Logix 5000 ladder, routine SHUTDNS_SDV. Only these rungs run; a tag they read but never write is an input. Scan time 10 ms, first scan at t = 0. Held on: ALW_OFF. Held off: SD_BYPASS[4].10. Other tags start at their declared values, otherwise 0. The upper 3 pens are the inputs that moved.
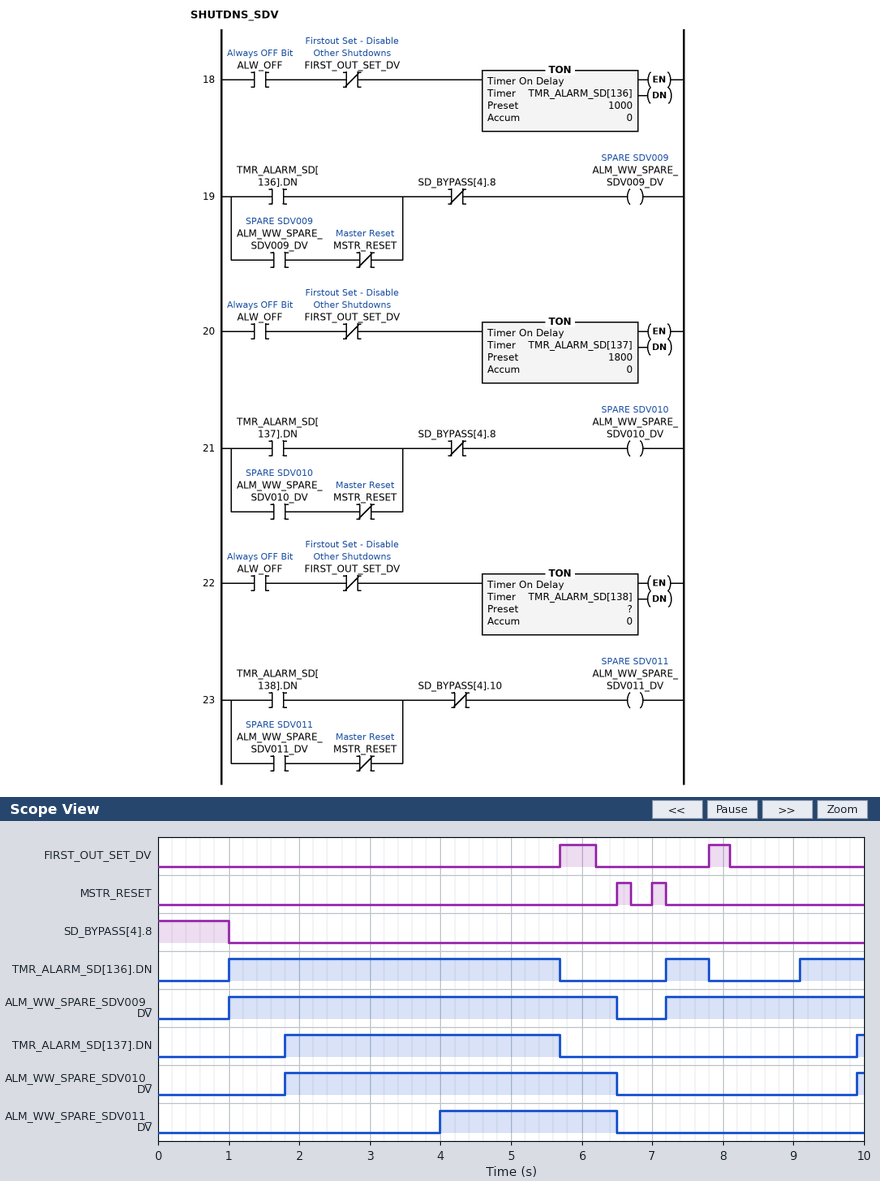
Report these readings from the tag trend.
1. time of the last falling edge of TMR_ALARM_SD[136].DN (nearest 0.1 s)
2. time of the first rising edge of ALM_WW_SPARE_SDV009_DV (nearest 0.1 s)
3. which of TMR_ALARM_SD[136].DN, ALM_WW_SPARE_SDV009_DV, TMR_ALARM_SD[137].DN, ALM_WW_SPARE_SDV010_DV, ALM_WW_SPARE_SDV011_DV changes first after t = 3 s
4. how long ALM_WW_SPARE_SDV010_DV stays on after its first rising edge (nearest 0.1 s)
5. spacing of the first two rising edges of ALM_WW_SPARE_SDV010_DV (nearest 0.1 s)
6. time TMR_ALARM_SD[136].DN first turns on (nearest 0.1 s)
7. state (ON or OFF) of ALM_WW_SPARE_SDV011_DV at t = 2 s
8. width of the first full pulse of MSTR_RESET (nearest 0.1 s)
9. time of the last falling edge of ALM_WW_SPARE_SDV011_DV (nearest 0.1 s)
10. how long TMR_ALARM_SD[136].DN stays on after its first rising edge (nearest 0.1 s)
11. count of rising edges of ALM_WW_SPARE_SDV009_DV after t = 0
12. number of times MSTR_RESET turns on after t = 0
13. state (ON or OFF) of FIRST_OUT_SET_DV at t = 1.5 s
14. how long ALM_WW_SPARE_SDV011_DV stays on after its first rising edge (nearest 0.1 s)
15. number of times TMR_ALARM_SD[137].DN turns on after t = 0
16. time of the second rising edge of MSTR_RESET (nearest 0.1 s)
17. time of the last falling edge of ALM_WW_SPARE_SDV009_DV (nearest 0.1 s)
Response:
7.8 s
1.0 s
ALM_WW_SPARE_SDV011_DV
4.7 s
8.1 s
1.0 s
OFF
0.2 s
6.5 s
4.7 s
2
2
OFF
2.5 s
2
7.0 s
6.5 s
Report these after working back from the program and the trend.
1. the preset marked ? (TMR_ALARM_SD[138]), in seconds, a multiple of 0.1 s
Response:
4.0 s
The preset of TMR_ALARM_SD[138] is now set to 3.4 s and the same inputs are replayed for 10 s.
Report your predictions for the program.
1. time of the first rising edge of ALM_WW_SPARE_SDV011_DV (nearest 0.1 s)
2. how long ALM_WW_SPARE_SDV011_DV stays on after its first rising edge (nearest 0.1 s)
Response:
3.4 s
3.1 s
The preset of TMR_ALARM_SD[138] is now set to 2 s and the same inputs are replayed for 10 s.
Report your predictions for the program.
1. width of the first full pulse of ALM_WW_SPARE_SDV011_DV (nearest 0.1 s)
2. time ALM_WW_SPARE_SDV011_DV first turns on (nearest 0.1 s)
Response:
4.5 s
2.0 s
